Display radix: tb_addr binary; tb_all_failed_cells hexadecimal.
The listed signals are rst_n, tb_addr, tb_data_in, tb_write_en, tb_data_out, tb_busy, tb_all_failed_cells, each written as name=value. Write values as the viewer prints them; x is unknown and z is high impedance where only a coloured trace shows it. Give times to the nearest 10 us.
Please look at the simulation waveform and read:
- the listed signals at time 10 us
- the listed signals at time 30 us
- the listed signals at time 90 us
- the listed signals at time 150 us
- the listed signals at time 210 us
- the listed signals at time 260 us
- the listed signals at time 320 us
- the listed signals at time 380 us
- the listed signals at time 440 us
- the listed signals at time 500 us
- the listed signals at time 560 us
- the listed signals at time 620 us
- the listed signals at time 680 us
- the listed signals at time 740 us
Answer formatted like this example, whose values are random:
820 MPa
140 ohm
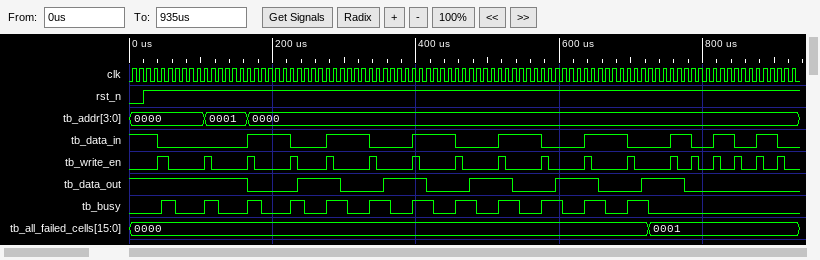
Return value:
rst_n=0, tb_addr=0000, tb_data_in=1, tb_write_en=0, tb_data_out=1, tb_busy=0, tb_all_failed_cells=0000
rst_n=1, tb_addr=0000, tb_data_in=1, tb_write_en=0, tb_data_out=1, tb_busy=0, tb_all_failed_cells=0000
rst_n=1, tb_addr=0000, tb_data_in=0, tb_write_en=0, tb_data_out=1, tb_busy=0, tb_all_failed_cells=0000
rst_n=1, tb_addr=0001, tb_data_in=0, tb_write_en=0, tb_data_out=1, tb_busy=0, tb_all_failed_cells=0000
rst_n=1, tb_addr=0000, tb_data_in=1, tb_write_en=0, tb_data_out=0, tb_busy=0, tb_all_failed_cells=0000
rst_n=1, tb_addr=0000, tb_data_in=0, tb_write_en=0, tb_data_out=1, tb_busy=0, tb_all_failed_cells=0000
rst_n=1, tb_addr=0000, tb_data_in=1, tb_write_en=0, tb_data_out=0, tb_busy=0, tb_all_failed_cells=0000
rst_n=1, tb_addr=0000, tb_data_in=0, tb_write_en=0, tb_data_out=1, tb_busy=0, tb_all_failed_cells=0000
rst_n=1, tb_addr=0000, tb_data_in=1, tb_write_en=0, tb_data_out=0, tb_busy=0, tb_all_failed_cells=0000
rst_n=1, tb_addr=0000, tb_data_in=0, tb_write_en=0, tb_data_out=1, tb_busy=0, tb_all_failed_cells=0000
rst_n=1, tb_addr=0000, tb_data_in=1, tb_write_en=0, tb_data_out=0, tb_busy=0, tb_all_failed_cells=0000
rst_n=1, tb_addr=0000, tb_data_in=0, tb_write_en=0, tb_data_out=1, tb_busy=0, tb_all_failed_cells=0000
rst_n=1, tb_addr=0000, tb_data_in=1, tb_write_en=0, tb_data_out=0, tb_busy=0, tb_all_failed_cells=0000
rst_n=1, tb_addr=0000, tb_data_in=0, tb_write_en=0, tb_data_out=1, tb_busy=0, tb_all_failed_cells=0001
